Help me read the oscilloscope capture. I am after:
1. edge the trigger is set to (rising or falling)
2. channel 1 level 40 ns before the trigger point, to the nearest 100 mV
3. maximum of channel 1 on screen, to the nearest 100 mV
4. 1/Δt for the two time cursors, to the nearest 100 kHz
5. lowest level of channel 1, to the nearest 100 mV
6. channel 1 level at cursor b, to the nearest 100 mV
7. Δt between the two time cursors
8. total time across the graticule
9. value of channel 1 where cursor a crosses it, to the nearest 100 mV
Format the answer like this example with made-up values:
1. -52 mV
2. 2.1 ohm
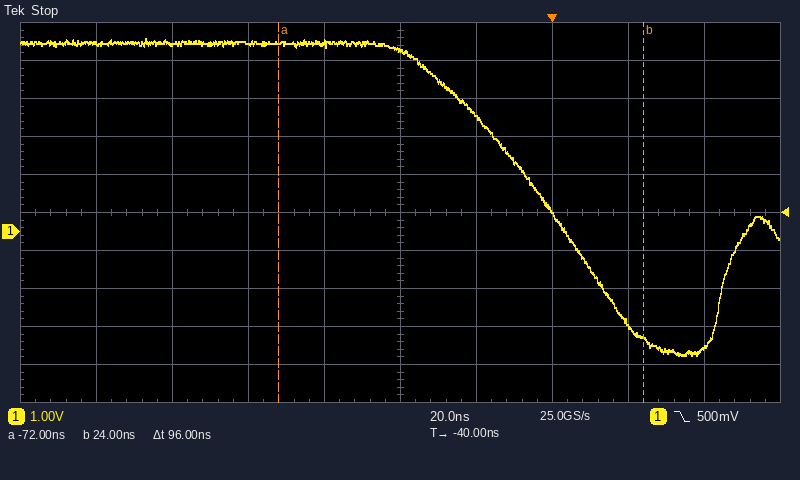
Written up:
1. falling
2. 4.8 V
3. 5.1 V
4. 10.4 MHz
5. -3.3 V
6. -2.8 V
7. 96 ns
8. 200 ns
9. 5.0 V
